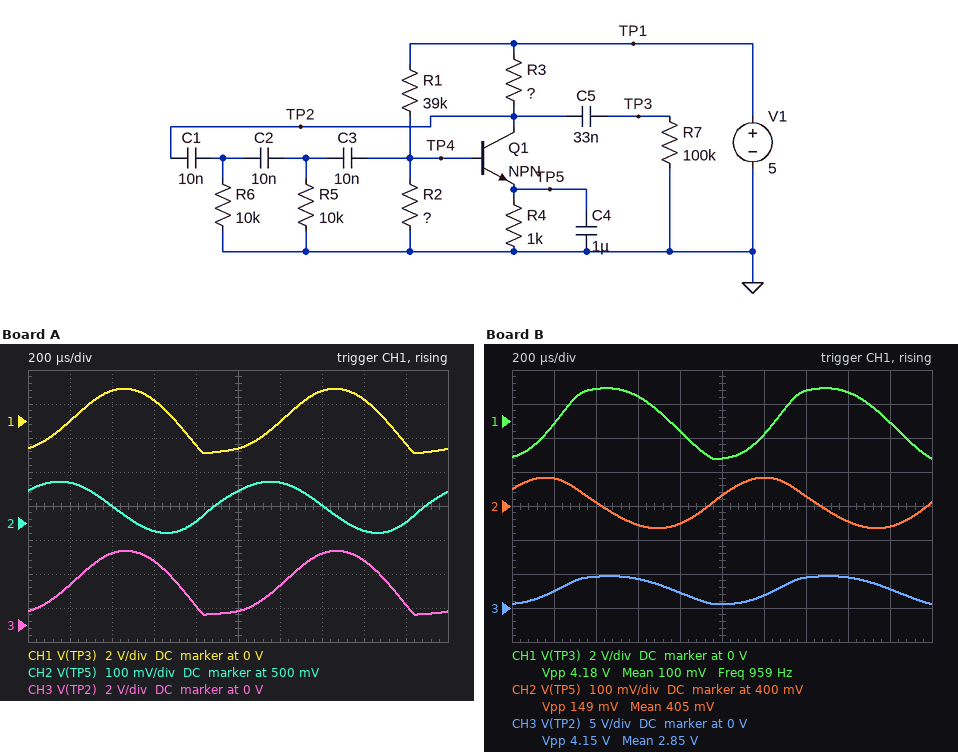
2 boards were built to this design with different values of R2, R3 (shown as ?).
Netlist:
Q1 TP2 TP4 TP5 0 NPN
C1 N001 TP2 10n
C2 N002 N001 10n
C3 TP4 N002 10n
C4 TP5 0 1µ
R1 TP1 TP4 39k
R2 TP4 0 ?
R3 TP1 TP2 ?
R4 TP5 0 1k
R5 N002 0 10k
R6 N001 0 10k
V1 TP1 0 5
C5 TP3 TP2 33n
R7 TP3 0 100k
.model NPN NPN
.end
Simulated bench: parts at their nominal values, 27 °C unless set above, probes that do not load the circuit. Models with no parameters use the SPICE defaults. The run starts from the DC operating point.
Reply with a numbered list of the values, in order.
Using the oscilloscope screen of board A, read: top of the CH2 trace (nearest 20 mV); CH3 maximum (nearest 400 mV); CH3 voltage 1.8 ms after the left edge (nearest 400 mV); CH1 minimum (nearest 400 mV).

1. 620 mV
2. 4.4 V
3. 1.2 V
4. -2.0 V
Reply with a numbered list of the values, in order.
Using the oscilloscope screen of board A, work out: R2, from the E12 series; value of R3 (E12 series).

1. 15 kΩ
2. 4.7 kΩ
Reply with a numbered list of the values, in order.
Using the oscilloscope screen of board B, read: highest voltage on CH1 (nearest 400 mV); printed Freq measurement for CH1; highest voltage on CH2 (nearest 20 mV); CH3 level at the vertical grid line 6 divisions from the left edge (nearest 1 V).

1. 2.0 V
2. 959 Hz
3. 480 mV
4. 2 V
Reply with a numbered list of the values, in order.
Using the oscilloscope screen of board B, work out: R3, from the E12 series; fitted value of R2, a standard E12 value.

1. 5.6 kΩ
2. 12 kΩ
